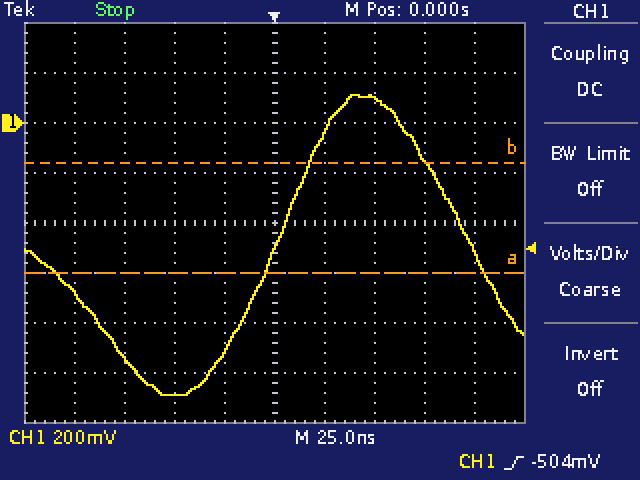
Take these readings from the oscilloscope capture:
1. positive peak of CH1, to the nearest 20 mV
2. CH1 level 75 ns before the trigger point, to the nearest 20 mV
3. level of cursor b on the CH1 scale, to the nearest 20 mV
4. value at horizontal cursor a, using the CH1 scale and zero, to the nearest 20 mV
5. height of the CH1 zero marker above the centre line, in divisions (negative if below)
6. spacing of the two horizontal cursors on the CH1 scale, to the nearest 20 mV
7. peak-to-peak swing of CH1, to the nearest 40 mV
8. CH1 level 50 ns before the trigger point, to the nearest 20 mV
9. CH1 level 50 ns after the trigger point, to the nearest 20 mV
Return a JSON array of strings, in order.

["120 mV", "-940 mV", "-160 mV", "-600 mV", "+2.0 div", "440 mV", "1.20 V", "-1.08 V", "100 mV"]
